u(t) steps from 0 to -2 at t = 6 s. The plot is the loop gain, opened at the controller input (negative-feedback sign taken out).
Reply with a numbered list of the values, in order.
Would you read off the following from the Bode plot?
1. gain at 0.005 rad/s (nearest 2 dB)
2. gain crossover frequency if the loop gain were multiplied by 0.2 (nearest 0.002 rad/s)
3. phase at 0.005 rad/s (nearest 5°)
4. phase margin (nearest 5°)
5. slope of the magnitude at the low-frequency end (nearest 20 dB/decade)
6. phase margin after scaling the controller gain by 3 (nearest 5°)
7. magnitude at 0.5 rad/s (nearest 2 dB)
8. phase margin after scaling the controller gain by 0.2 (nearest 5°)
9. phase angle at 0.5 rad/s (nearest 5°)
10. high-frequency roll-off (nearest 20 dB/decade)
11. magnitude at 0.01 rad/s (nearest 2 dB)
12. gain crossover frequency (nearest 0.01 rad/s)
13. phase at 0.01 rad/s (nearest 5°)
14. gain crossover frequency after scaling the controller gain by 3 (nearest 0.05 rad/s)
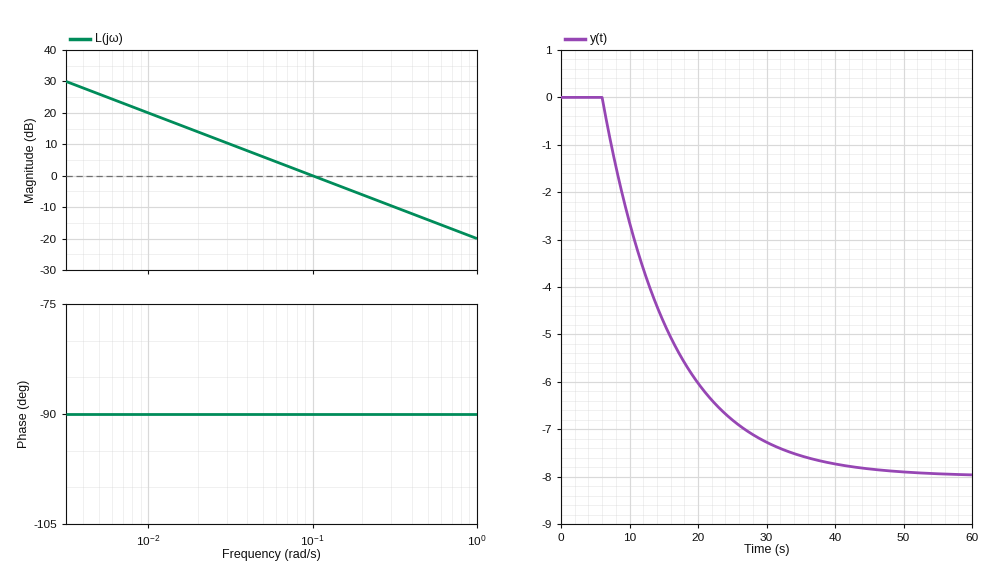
1. 26 dB
2. 0.020 rad/s
3. -90°
4. 90°
5. -20 dB/decade
6. 90°
7. -14 dB
8. 90°
9. -90°
10. -20 dB/decade
11. 20 dB
12. 0.10 rad/s
13. -90°
14. 0.30 rad/s
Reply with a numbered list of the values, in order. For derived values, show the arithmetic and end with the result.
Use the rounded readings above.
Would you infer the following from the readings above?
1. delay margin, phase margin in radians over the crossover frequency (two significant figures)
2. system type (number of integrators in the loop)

1. 90 × π / 180 / 0.1 = 16 s
2. 1
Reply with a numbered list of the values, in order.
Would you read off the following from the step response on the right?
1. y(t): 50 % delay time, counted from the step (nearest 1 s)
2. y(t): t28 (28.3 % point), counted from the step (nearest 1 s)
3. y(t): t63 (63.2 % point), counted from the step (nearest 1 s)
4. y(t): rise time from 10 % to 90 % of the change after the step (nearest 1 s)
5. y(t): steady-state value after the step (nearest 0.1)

1. 7 s
2. 3 s
3. 10 s
4. 22 s
5. -8.0
